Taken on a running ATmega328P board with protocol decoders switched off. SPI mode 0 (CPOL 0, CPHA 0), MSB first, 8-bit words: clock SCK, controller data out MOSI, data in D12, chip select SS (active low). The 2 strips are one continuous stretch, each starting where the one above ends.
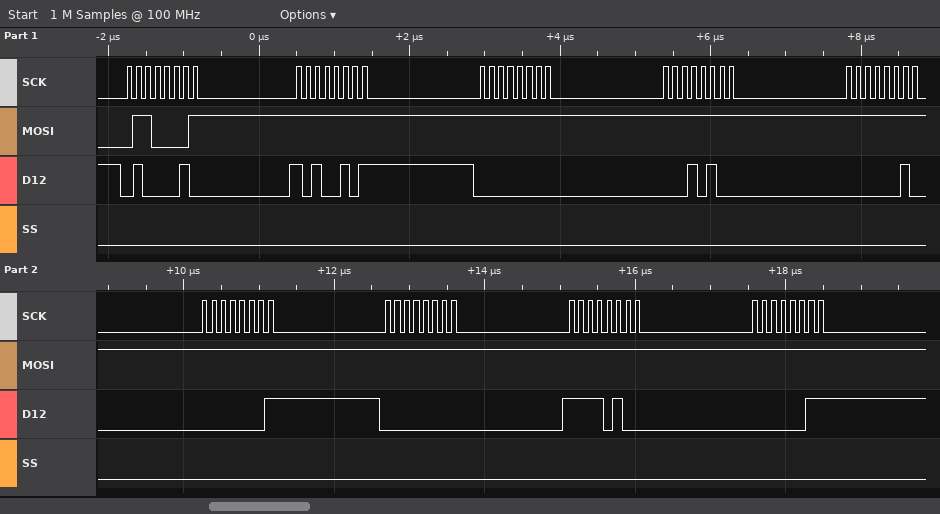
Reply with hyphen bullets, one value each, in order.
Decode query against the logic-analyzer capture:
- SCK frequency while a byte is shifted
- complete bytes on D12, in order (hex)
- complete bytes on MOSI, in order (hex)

- 8 MHz
- 0x42 0xA5 0x00 0x14 0x02 0x01 0x00 0xF4 0x03
- 0x61 0xFF 0xFF 0xFF 0xFF 0xFF 0xFF 0xFF 0xFF
